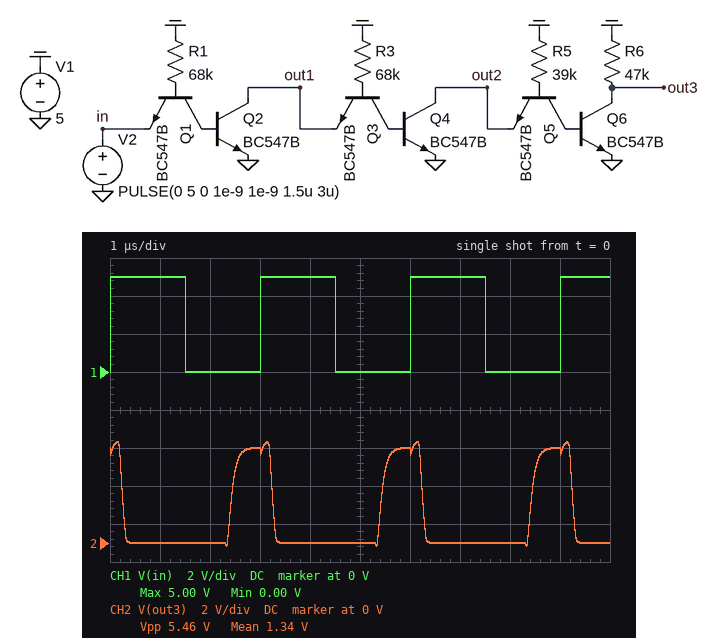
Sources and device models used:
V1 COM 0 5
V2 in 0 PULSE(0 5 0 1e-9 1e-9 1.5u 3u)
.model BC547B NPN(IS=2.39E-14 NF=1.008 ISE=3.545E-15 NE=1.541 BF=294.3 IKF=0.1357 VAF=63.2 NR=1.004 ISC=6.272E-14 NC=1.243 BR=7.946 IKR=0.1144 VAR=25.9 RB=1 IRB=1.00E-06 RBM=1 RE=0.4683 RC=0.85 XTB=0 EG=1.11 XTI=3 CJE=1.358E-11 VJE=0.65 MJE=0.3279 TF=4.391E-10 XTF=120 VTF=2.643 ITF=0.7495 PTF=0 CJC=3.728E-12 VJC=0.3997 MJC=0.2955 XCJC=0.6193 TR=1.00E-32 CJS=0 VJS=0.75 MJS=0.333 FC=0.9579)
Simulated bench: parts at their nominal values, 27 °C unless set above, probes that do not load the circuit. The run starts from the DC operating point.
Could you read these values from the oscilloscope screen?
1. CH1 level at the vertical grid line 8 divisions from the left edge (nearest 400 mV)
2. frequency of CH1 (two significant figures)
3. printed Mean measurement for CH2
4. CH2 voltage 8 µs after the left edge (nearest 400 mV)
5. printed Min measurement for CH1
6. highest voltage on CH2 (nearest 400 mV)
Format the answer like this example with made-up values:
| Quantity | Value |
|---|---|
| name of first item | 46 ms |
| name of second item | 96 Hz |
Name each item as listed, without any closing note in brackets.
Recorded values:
| Quantity | Value |
|---|---|
| CH1 level at the vertical grid line 8 divisions from the left edge | 0 V |
| frequency of CH1 | 330 kHz |
| printed Mean measurement for CH2 | 1.34 V |
| CH2 voltage 8 µs after the left edge | 0 V |
| printed Min measurement for CH1 | 0.00 V |
| highest voltage on CH2 | 5.2 V |
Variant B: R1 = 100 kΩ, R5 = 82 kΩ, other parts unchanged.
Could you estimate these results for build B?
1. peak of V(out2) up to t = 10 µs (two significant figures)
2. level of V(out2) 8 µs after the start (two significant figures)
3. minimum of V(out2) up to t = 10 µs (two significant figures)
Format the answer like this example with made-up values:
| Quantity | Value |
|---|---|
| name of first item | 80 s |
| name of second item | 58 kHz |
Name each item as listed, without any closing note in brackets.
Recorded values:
| Quantity | Value |
|---|---|
| peak of V(out2) up to t = 10 µs | 620 mV |
| level of V(out2) 8 µs after the start | 610 mV |
| minimum of V(out2) up to t = 10 µs | -400 mV |
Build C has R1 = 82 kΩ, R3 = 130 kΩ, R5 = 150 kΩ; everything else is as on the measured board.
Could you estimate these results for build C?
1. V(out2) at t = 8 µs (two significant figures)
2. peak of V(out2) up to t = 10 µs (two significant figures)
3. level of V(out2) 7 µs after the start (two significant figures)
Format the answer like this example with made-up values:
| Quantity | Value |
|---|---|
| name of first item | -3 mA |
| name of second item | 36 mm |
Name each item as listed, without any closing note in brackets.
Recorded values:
| Quantity | Value |
|---|---|
| V(out2) at t = 8 µs | 600 mV |
| peak of V(out2) up to t = 10 µs | 610 mV |
| level of V(out2) 7 µs after the start | 580 mV |
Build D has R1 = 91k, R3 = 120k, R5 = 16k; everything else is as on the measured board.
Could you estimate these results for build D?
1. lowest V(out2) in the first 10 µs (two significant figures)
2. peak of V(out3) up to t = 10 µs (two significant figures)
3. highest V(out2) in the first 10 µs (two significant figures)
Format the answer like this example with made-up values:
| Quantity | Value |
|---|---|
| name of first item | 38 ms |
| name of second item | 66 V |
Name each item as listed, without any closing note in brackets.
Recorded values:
| Quantity | Value |
|---|---|
| lowest V(out2) in the first 10 µs | -290 mV |
| peak of V(out3) up to t = 10 µs | 5.4 V |
| highest V(out2) in the first 10 µs | 650 mV |
